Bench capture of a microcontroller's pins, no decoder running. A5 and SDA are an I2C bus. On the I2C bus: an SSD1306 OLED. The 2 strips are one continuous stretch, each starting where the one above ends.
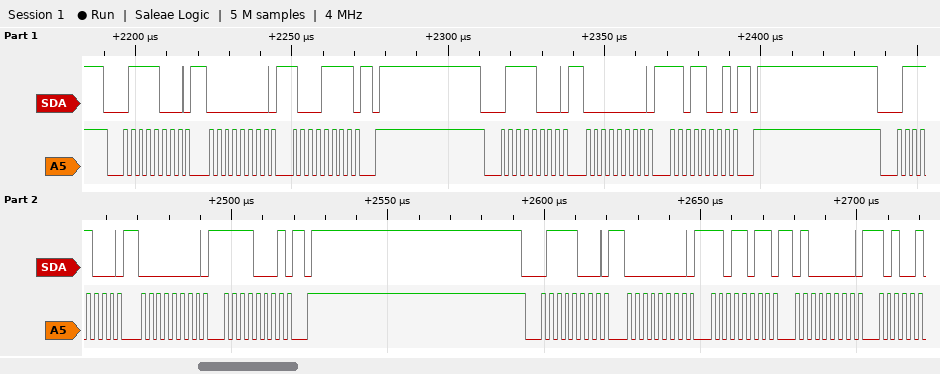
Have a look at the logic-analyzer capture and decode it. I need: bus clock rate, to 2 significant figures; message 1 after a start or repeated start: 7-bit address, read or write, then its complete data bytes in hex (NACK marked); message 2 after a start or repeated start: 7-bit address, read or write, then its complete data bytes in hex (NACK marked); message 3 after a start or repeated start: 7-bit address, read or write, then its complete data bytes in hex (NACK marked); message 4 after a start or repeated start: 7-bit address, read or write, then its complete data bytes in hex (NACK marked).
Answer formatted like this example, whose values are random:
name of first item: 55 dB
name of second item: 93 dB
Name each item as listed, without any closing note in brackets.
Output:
bus clock rate, to 2 significant figures: 400 kHz
message 1 after a start or repeated start: 7-bit address, read or write, then its complete data bytes in hex: 0x3C write: 00 8F
message 2 after a start or repeated start: 7-bit address, read or write, then its complete data bytes in hex: 0x3C write: 00 D9
message 3 after a start or repeated start: 7-bit address, read or write, then its complete data bytes in hex: 0x3C write: 00 F1
message 4 after a start or repeated start: 7-bit address, read or write, then its complete data bytes in hex: 0x3C write: 00 DB 40
